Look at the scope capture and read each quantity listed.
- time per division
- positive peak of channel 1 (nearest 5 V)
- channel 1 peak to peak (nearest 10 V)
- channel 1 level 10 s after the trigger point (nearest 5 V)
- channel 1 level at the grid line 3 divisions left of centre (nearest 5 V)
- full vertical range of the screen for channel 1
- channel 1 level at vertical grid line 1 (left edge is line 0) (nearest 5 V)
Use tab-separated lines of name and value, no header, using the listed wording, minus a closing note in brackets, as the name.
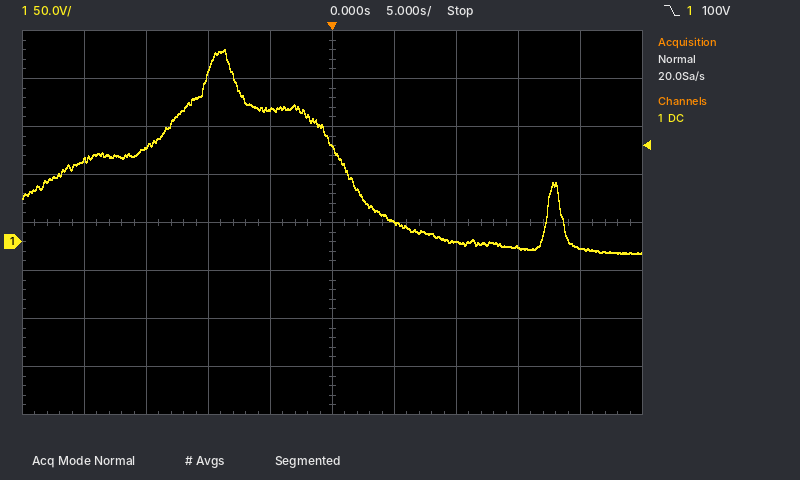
time per division	5 s
positive peak of channel 1	200 V
channel 1 peak to peak	210 V
channel 1 level 10 s after the trigger point	0 V
channel 1 level at the grid line 3 divisions left of centre	100 V
full vertical range of the screen for channel 1	400 V
channel 1 level at vertical grid line 1 (left edge is line 0)	85 V
